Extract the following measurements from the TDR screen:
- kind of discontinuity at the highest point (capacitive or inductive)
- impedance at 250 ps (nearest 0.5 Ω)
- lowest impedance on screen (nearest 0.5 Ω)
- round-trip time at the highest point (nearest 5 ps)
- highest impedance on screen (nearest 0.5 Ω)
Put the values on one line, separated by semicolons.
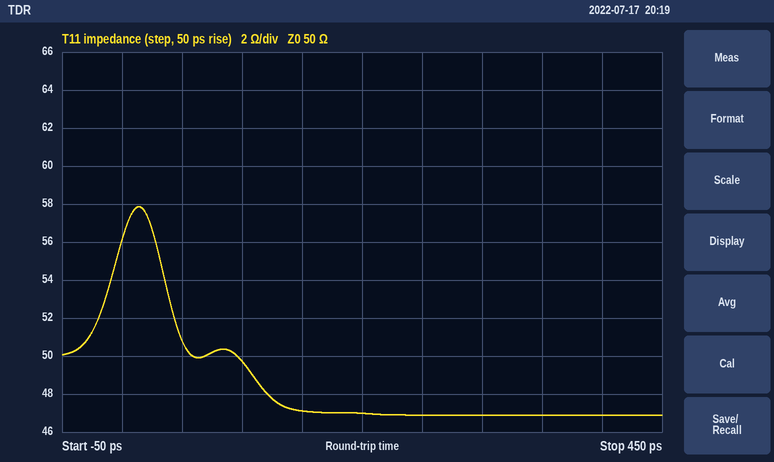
inductive; 47.0 Ω; 47.0 Ω; 15 ps; 58.0 Ω
